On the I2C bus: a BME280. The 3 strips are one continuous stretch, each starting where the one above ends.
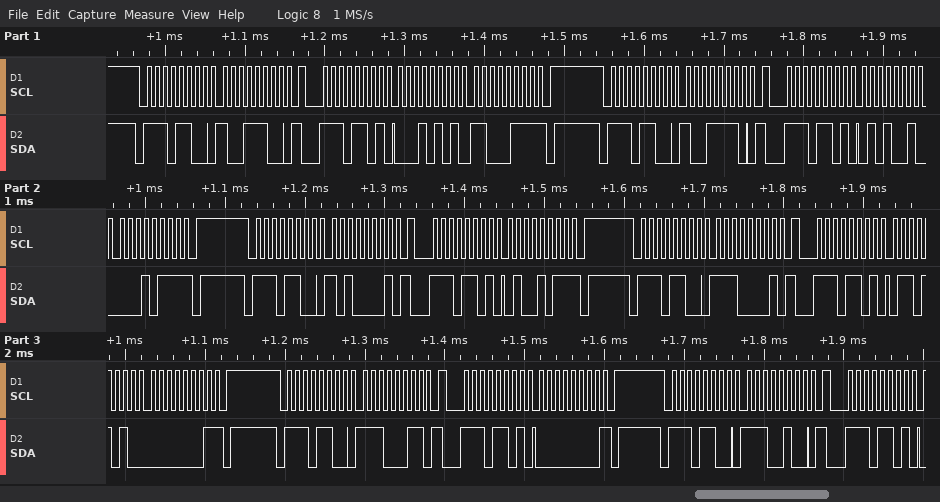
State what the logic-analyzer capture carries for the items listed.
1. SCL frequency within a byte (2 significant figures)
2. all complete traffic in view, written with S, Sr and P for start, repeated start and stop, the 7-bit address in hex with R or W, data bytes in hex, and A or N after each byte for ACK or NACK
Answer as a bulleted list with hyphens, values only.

- 100 kHz
- S 76W A 9C A Sr 76R A 15 A C7 N P S 76W A 9E A Sr 76R A 52 A 17 N P S 76W A A1 A Sr 76R A 4B N P S 76W A E1 A Sr 76R A 6A A 01 N P S 76W A E3 A Sr 76R A 00 N P S 76W A E4 A Sr 76R A
